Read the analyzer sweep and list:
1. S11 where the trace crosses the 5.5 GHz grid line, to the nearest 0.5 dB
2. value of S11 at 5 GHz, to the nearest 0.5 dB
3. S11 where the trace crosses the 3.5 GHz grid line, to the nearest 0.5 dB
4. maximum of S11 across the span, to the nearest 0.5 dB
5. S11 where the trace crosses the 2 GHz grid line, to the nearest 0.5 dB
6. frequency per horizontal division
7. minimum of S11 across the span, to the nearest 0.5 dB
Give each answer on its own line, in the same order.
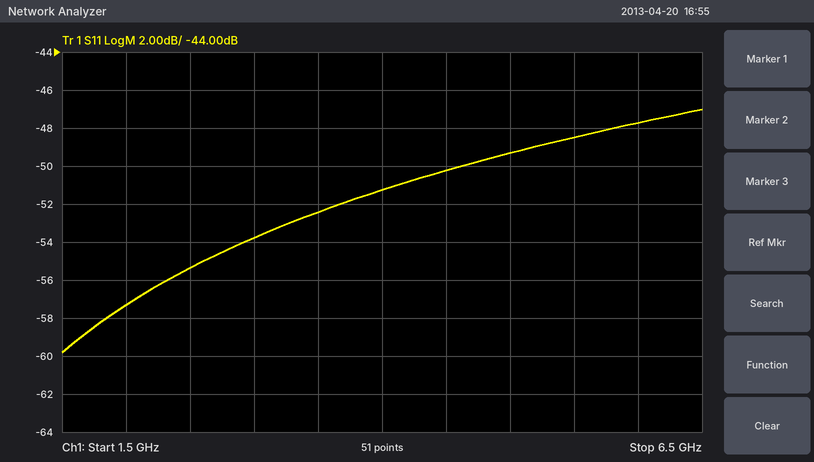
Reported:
-48.5 dB
-49.5 dB
-52.5 dB
-47.0 dB
-57.5 dB
500 MHz
-60.0 dB
